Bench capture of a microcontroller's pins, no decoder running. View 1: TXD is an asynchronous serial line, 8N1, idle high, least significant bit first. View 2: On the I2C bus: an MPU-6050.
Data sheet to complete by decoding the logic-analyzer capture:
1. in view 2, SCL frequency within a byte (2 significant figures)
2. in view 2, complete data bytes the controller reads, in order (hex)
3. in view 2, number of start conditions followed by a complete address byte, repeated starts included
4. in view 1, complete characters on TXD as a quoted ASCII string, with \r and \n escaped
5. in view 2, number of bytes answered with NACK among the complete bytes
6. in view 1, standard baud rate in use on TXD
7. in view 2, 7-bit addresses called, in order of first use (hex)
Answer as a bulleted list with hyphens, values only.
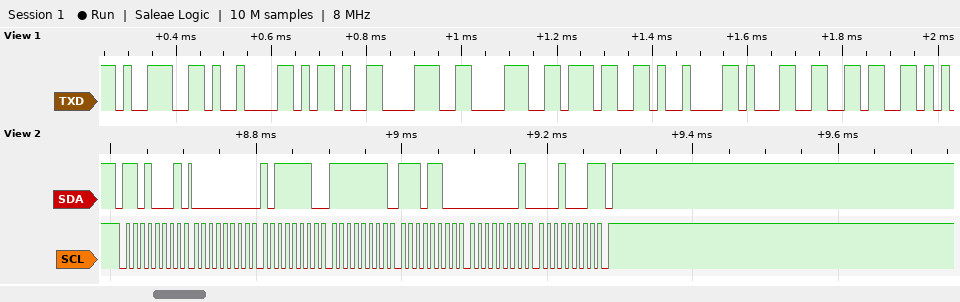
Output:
- 100 kHz
- 00 BE FF EC 01 11
- 1
- "9\t-887\t16"
- 1
- 57600 baud
- 0x68
